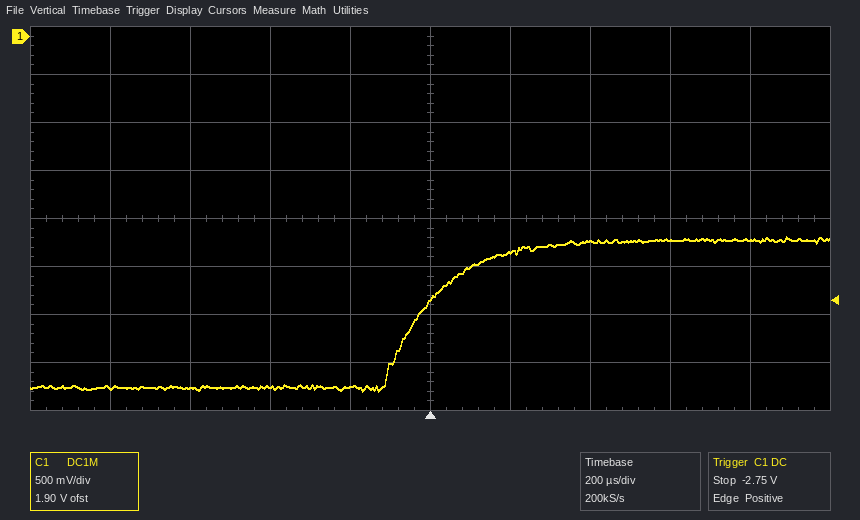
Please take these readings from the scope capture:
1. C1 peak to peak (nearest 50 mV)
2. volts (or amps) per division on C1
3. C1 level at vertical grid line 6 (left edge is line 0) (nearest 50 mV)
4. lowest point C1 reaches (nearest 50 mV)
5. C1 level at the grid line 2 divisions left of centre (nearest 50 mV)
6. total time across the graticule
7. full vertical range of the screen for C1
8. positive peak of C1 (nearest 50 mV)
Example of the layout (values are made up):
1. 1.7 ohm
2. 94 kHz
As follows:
1. 1.60 V
2. 500 mV
3. -2.25 V
4. -3.70 V
5. -3.65 V
6. 2 ms
7. 4 V
8. -2.10 V
